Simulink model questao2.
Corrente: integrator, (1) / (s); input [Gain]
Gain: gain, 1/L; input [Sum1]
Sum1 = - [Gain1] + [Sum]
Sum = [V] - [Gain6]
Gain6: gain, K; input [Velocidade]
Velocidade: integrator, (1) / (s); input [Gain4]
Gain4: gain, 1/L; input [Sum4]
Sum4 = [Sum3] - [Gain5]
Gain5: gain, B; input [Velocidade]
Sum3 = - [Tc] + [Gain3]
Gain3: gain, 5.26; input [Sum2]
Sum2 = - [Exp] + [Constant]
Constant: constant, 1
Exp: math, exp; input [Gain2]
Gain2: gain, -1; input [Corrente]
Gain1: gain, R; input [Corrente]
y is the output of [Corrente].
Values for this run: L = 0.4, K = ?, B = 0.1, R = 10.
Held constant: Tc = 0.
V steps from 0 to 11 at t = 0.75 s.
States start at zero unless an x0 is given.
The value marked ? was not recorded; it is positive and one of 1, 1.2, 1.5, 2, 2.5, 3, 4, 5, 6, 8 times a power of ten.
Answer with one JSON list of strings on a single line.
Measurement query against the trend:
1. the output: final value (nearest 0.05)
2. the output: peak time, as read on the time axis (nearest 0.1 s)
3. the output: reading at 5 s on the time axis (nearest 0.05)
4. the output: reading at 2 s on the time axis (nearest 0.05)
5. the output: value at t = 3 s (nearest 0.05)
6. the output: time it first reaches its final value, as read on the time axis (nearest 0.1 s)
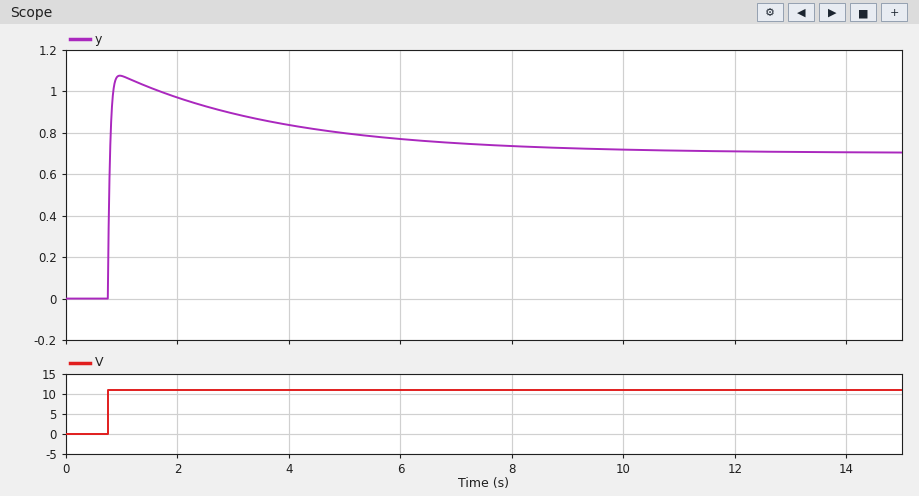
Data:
["0.70", "1.0 s", "0.80", "0.95", "0.90", "0.8 s"]
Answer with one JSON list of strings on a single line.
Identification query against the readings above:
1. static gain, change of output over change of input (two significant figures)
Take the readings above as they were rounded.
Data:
["0.064"]
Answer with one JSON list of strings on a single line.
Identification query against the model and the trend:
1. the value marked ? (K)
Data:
["0.15"]
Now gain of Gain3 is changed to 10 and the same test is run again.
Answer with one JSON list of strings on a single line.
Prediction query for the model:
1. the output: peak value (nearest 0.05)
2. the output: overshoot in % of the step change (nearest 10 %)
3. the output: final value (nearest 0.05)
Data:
["1.05", "110 %", "0.50"]
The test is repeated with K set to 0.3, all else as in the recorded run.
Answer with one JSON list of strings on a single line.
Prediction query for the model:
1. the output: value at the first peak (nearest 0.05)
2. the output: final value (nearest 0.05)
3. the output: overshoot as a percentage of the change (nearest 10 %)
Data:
["1.05", "0.50", "120 %"]
